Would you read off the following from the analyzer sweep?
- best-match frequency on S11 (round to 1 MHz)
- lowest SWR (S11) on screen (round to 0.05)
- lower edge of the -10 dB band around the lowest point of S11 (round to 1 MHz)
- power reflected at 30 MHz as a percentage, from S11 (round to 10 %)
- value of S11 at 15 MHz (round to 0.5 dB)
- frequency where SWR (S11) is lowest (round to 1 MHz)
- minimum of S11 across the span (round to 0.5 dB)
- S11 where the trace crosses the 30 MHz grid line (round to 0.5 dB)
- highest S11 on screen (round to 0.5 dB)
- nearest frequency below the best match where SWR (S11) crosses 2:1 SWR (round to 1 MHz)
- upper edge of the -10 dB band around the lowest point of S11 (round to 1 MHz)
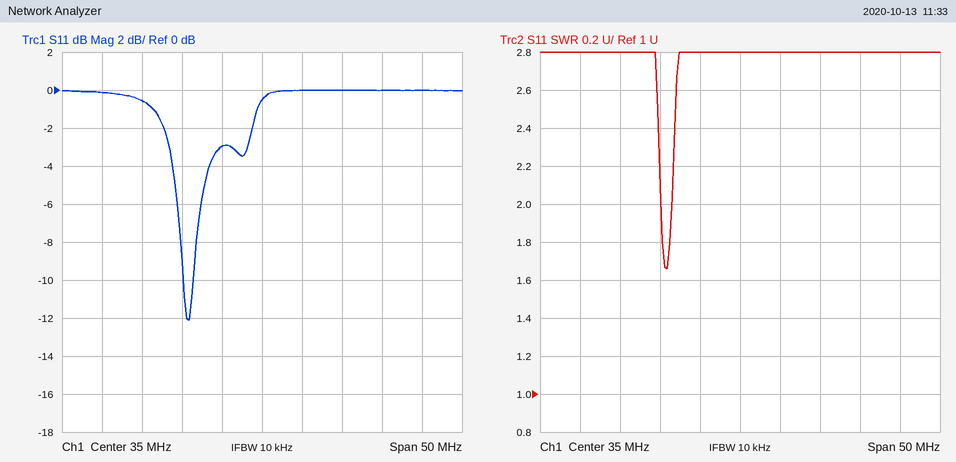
26 MHz
1.65
25 MHz
50 %
0.0 dB
26 MHz
-12.0 dB
-3.0 dB
0.0 dB
25 MHz
26 MHz
